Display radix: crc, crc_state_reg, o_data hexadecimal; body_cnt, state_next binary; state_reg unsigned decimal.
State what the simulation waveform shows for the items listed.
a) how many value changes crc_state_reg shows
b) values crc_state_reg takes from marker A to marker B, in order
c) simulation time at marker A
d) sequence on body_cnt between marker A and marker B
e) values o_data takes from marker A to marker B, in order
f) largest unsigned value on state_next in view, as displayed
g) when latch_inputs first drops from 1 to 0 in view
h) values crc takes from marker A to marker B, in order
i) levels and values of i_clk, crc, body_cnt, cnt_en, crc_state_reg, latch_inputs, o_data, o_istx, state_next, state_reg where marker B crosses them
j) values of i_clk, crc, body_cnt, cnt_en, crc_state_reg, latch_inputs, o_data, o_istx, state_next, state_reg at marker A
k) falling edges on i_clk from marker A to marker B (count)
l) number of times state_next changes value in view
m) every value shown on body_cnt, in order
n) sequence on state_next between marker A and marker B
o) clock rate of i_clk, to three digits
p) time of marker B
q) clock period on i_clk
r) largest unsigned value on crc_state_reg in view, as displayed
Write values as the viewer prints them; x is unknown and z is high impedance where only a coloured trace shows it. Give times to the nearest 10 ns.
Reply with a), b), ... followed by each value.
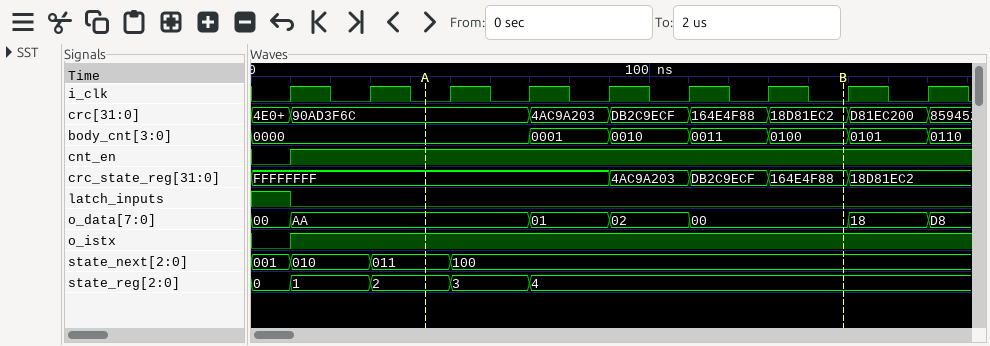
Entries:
a) 4
b) FFFFFFFF, 4AC9A203, DB2C9ECF, 164E4F88
c) 40 ns
d) 0000, 0001, 0010, 0011, 0100
e) AA, 01, 02, 00
f) 100
g) 10 ns
h) 90AD3F6C, 4AC9A203, DB2C9ECF, 164E4F88, 18D81EC2
i) i_clk=0, crc=18D81EC2, body_cnt=0100, cnt_en=1, crc_state_reg=164E4F88, latch_inputs=0, o_data=00, o_istx=1, state_next=100, state_reg=4
j) i_clk=0, crc=90AD3F6C, body_cnt=0000, cnt_en=1, crc_state_reg=FFFFFFFF, latch_inputs=0, o_data=AA, o_istx=1, state_next=011, state_reg=2
k) 5
l) 3
m) 0000, 0001, 0010, 0011, 0100, 0101, 0110
n) 011, 100
o) 50.0 MHz
p) 150 ns
q) 20 ns
r) FFFFFFFF
